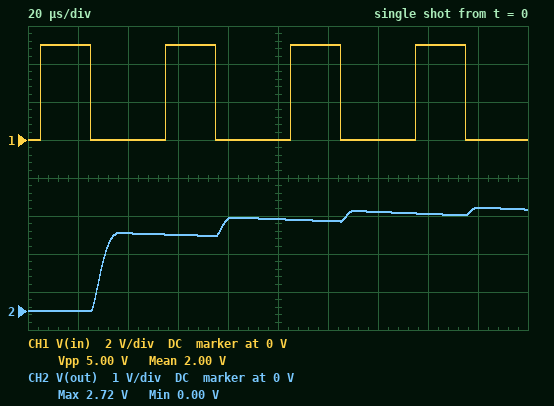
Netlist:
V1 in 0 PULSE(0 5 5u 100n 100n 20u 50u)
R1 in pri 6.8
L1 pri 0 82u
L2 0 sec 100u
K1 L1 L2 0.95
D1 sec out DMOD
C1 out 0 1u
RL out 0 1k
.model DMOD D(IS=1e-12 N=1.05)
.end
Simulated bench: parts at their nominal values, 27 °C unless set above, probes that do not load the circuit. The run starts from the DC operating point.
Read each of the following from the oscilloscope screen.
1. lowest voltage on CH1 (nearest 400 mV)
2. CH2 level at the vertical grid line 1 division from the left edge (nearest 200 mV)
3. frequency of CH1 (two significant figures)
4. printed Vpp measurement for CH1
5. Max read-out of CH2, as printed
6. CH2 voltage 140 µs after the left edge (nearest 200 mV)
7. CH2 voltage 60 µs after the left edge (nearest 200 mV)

0 V
0 V
20 kHz
5.00 V
2.72 V
2.6 V
2.0 V
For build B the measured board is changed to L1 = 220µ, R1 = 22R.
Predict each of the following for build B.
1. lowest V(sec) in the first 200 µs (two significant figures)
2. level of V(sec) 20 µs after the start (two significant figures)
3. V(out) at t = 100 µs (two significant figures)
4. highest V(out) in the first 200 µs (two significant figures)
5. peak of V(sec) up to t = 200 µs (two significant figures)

-3.2 V
-720 mV
1.2 V
1.4 V
2.1 V
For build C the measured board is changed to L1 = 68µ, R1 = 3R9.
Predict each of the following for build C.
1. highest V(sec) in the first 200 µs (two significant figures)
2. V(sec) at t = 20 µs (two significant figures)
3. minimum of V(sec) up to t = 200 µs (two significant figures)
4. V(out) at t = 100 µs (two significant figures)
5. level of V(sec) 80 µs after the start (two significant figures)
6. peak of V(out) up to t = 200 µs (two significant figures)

3.5 V
-2.4 V
-5.7 V
2.7 V
3.4 V
2.9 V
